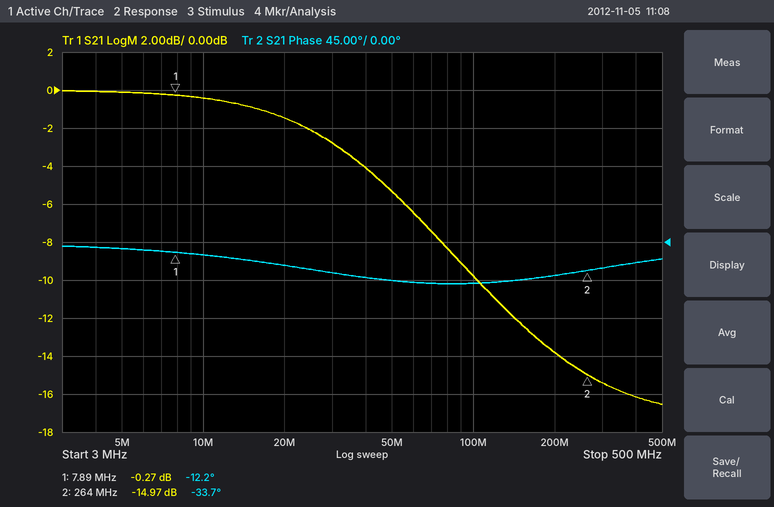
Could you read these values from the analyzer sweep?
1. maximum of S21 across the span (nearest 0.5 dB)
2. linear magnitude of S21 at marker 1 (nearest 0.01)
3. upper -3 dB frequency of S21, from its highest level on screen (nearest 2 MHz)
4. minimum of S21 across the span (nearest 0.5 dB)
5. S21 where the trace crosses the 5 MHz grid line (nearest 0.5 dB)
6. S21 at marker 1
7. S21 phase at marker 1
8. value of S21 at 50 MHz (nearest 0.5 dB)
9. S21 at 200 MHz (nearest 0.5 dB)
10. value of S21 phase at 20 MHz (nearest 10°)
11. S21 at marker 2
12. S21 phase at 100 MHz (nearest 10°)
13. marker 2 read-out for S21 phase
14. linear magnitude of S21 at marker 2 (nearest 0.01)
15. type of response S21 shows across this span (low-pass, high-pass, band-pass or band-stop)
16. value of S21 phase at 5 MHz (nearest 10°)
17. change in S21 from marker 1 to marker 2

0.0 dB
0.97
32 MHz
-16.5 dB
0.0 dB
-0.27 dB
-12.2°
-5.5 dB
-14.0 dB
-30°
-14.97 dB
-50°
-33.7°
0.18
low-pass
-10°
-14.70 dB
